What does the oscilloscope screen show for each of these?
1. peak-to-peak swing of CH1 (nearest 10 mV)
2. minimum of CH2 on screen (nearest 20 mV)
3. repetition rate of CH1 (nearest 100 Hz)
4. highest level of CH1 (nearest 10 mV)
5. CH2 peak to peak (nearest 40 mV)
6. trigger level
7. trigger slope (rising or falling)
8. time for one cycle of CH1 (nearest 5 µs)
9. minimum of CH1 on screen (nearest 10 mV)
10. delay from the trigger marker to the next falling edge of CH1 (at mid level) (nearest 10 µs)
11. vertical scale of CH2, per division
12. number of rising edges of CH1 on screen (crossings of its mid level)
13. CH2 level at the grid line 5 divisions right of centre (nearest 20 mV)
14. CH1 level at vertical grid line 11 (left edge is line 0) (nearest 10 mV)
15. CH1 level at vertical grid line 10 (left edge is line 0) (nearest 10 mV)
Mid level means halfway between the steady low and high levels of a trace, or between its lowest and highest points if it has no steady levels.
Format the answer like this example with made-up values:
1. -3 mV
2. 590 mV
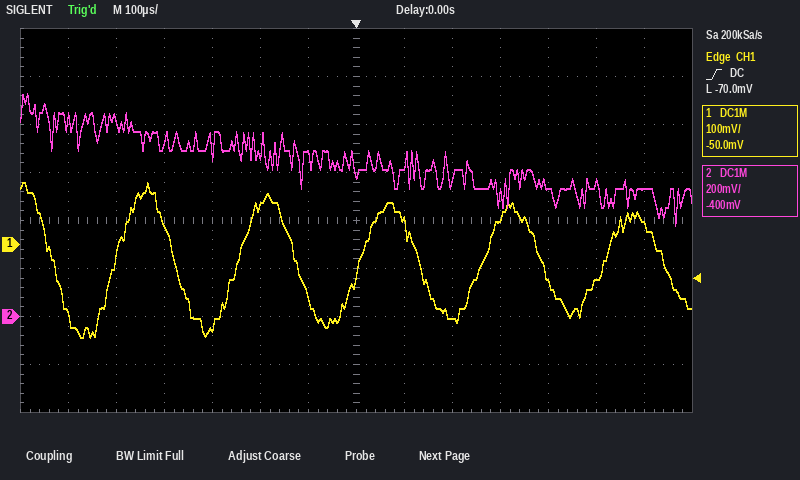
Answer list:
1. 320 mV
2. 380 mV
3. 3.9 kHz
4. 130 mV
5. 560 mV
6. -70.0 mV
7. rising
8. 255 µs
9. -190 mV
10. 130 µs
11. 200 mV
12. 5
13. 560 mV
14. -80 mV
15. 50 mV
